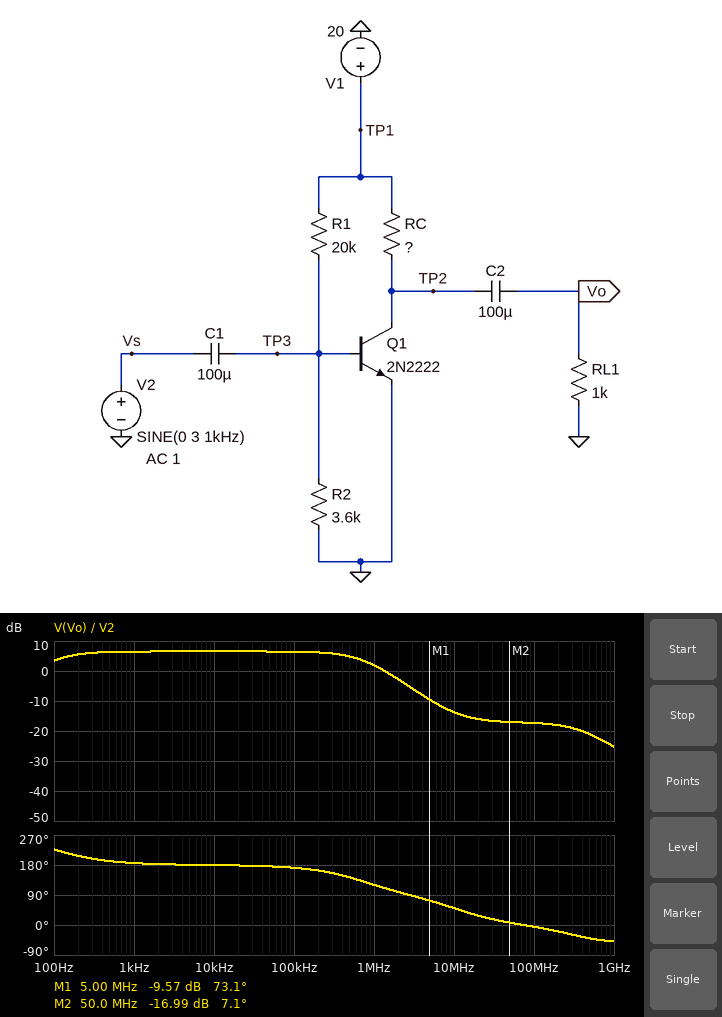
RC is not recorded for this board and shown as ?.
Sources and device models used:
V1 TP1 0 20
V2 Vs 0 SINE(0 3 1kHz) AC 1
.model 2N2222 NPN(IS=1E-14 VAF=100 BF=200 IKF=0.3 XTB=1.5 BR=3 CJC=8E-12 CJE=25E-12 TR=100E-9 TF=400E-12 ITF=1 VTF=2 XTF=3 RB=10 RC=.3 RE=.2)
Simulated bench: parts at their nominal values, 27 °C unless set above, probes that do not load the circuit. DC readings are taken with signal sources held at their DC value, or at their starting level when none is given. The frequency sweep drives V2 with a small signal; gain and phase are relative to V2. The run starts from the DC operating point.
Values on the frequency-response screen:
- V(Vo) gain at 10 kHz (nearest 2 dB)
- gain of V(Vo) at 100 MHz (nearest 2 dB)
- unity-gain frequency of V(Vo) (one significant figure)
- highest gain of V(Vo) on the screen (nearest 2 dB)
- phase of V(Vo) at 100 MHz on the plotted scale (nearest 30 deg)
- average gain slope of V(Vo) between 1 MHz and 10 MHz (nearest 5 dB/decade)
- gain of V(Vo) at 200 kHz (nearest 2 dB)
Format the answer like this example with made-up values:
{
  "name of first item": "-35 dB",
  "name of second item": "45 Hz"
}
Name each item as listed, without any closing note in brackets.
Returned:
{
  "V(Vo) gain at 10 kHz": "6 dB",
  "gain of V(Vo) at 100 MHz": "-18 dB",
  "unity-gain frequency of V(Vo)": "1 MHz",
  "highest gain of V(Vo) on the screen": "6 dB",
  "phase of V(Vo) at 100 MHz on the plotted scale": "0 deg",
  "average gain slope of V(Vo) between 1 MHz and 10 MHz": "-15 dB/decade",
  "gain of V(Vo) at 200 kHz": "6 dB"
}
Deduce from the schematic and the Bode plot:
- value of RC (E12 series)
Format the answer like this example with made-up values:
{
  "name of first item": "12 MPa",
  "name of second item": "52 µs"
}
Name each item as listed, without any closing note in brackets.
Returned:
{
  "value of RC": "1.2 kΩ"
}
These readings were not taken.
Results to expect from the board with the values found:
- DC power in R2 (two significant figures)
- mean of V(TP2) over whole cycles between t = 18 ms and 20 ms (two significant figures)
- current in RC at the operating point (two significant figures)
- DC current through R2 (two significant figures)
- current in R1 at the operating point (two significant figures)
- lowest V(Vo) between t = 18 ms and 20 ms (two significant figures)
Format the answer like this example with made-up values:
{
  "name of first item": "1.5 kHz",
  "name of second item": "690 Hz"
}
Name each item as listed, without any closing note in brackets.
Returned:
{
  "DC power in R2": "150 µW",
  "mean of V(TP2) over whole cycles between t = 18 ms and 20 ms": "8.2 V",
  "current in RC at the operating point": "17 mA",
  "DC current through R2": "210 µA",
  "current in R1 at the operating point": "960 µA",
  "lowest V(Vo) between t = 18 ms and 20 ms": "-1.3 V"
}
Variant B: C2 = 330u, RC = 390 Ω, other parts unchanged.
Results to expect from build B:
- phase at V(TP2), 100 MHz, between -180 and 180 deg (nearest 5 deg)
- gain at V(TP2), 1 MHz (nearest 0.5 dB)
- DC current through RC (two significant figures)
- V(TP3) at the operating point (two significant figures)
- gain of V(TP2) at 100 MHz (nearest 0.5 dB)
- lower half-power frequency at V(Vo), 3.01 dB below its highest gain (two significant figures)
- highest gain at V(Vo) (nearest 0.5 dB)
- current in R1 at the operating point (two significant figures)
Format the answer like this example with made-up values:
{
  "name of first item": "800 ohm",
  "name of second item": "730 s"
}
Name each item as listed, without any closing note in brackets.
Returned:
{
  "phase at V(TP2), 100 MHz, between -180 and 180 deg": "10 deg",
  "gain at V(TP2), 1 MHz": "7.5 dB",
  "DC current through RC": "51 mA",
  "V(TP3) at the operating point": "780 mV",
  "gain of V(TP2) at 100 MHz": "-22.5 dB",
  "lower half-power frequency at V(Vo), 3.01 dB below its highest gain": "130 Hz",
  "highest gain at V(Vo)": "13.0 dB",
  "current in R1 at the operating point": "960 µA"
}
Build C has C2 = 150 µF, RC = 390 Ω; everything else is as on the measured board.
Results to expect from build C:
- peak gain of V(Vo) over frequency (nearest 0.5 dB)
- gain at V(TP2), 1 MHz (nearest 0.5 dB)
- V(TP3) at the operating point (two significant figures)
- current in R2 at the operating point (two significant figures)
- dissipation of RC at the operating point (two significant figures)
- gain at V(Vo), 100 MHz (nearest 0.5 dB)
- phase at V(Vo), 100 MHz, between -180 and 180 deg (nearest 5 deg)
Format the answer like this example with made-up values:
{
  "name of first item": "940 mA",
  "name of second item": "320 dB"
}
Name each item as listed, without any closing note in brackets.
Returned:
{
  "peak gain of V(Vo) over frequency": "13.0 dB",
  "gain at V(TP2), 1 MHz": "7.5 dB",
  "V(TP3) at the operating point": "780 mV",
  "current in R2 at the operating point": "220 µA",
  "dissipation of RC at the operating point": "1.0 W",
  "gain at V(Vo), 100 MHz": "-22.5 dB",
  "phase at V(Vo), 100 MHz, between -180 and 180 deg": "10 deg"
}
